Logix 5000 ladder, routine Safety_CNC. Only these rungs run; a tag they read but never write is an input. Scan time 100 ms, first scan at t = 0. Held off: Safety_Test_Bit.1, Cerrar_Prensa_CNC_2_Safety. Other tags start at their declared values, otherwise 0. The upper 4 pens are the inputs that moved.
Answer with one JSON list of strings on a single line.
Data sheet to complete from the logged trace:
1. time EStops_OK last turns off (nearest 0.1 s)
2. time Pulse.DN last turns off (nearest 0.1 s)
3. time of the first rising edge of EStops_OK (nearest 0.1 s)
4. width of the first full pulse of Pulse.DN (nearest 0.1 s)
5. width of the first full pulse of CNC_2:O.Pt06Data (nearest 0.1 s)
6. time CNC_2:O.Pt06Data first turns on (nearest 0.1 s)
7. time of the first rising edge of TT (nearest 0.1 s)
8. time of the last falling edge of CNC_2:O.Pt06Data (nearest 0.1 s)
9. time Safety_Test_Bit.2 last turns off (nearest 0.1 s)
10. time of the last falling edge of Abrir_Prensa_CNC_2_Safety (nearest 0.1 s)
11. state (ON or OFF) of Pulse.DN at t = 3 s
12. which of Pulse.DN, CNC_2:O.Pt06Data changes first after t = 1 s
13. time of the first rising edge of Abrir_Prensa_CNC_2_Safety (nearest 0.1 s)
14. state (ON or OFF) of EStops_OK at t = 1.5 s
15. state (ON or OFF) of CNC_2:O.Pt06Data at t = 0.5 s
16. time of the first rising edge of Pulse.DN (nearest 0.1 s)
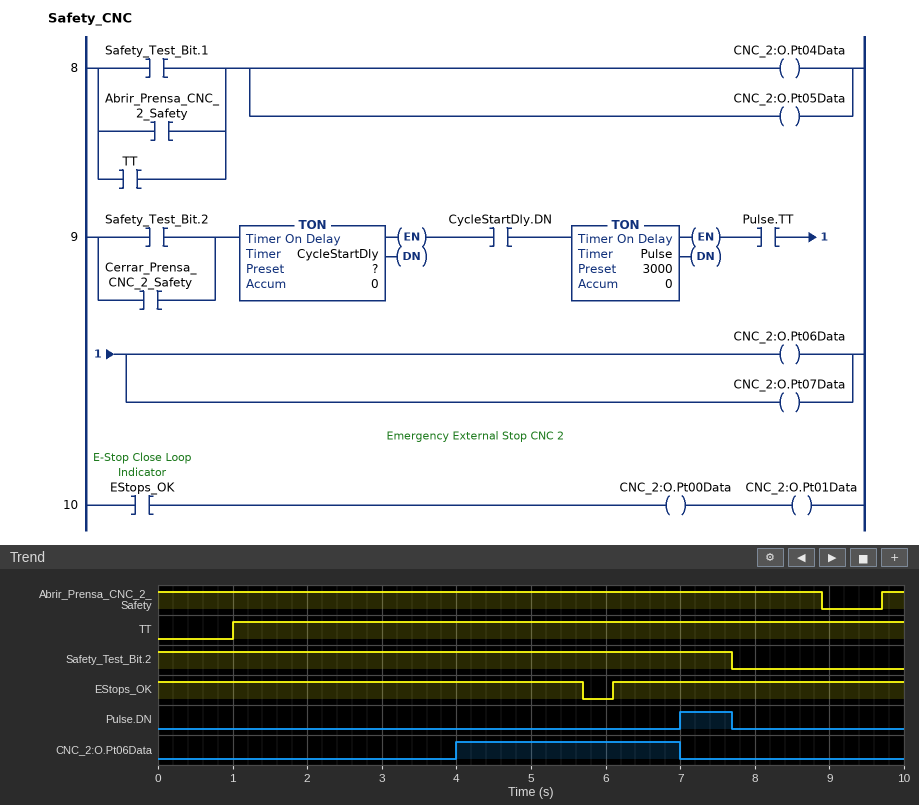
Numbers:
["5.7 s", "7.7 s", "6.1 s", "0.7 s", "3.0 s", "4.0 s", "1.0 s", "7.0 s", "7.7 s", "8.9 s", "OFF", "CNC_2:O.Pt06Data", "9.7 s", "ON", "OFF", "7.0 s"]
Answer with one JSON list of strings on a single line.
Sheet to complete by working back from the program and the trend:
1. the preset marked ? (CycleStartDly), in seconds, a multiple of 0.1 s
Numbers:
["4.0 s"]
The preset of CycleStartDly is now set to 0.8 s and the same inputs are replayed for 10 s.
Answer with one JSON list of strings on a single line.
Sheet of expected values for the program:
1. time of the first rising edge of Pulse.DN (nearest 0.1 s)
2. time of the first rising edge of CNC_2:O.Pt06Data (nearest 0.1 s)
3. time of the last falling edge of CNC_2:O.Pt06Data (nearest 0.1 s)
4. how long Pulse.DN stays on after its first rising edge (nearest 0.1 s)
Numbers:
["3.8 s", "0.8 s", "3.8 s", "3.9 s"]
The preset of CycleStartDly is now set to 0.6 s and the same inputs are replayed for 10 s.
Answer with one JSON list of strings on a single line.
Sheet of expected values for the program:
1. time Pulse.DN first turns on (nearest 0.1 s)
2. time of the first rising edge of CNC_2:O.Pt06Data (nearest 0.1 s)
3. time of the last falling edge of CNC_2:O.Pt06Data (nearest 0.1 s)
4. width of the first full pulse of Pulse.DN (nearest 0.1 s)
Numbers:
["3.6 s", "0.6 s", "3.6 s", "4.1 s"]
